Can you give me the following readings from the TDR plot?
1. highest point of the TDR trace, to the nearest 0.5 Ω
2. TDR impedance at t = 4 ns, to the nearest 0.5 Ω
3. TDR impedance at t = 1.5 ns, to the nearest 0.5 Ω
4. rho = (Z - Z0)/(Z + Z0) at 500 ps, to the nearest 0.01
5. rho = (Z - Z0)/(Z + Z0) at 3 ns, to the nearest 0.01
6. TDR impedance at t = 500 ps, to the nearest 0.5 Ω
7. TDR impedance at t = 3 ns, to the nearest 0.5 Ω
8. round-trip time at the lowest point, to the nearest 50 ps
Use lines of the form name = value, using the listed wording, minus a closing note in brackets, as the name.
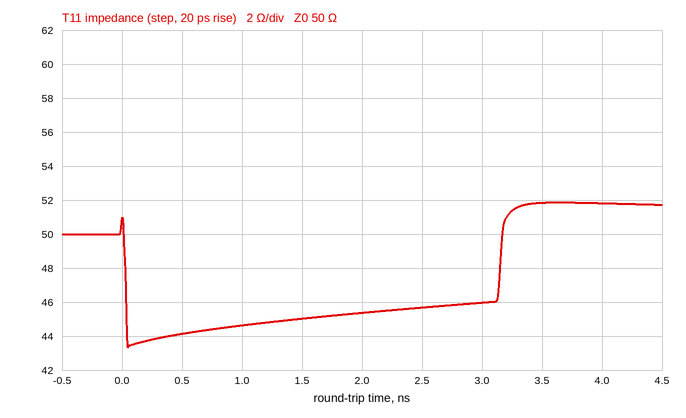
highest point of the TDR trace, to the nearest 0.5 Ω = 52.0 Ω
TDR impedance at t = 4 ns, to the nearest 0.5 Ω = 52.0 Ω
TDR impedance at t = 1.5 ns, to the nearest 0.5 Ω = 45.0 Ω
rho = (Z - Z0)/(Z + Z0) at 500 ps, to the nearest 0.01 = -0.06
rho = (Z - Z0)/(Z + Z0) at 3 ns, to the nearest 0.01 = -0.04
TDR impedance at t = 500 ps, to the nearest 0.5 Ω = 44.0 Ω
TDR impedance at t = 3 ns, to the nearest 0.5 Ω = 46.0 Ω
round-trip time at the lowest point, to the nearest 50 ps = 50 ps
